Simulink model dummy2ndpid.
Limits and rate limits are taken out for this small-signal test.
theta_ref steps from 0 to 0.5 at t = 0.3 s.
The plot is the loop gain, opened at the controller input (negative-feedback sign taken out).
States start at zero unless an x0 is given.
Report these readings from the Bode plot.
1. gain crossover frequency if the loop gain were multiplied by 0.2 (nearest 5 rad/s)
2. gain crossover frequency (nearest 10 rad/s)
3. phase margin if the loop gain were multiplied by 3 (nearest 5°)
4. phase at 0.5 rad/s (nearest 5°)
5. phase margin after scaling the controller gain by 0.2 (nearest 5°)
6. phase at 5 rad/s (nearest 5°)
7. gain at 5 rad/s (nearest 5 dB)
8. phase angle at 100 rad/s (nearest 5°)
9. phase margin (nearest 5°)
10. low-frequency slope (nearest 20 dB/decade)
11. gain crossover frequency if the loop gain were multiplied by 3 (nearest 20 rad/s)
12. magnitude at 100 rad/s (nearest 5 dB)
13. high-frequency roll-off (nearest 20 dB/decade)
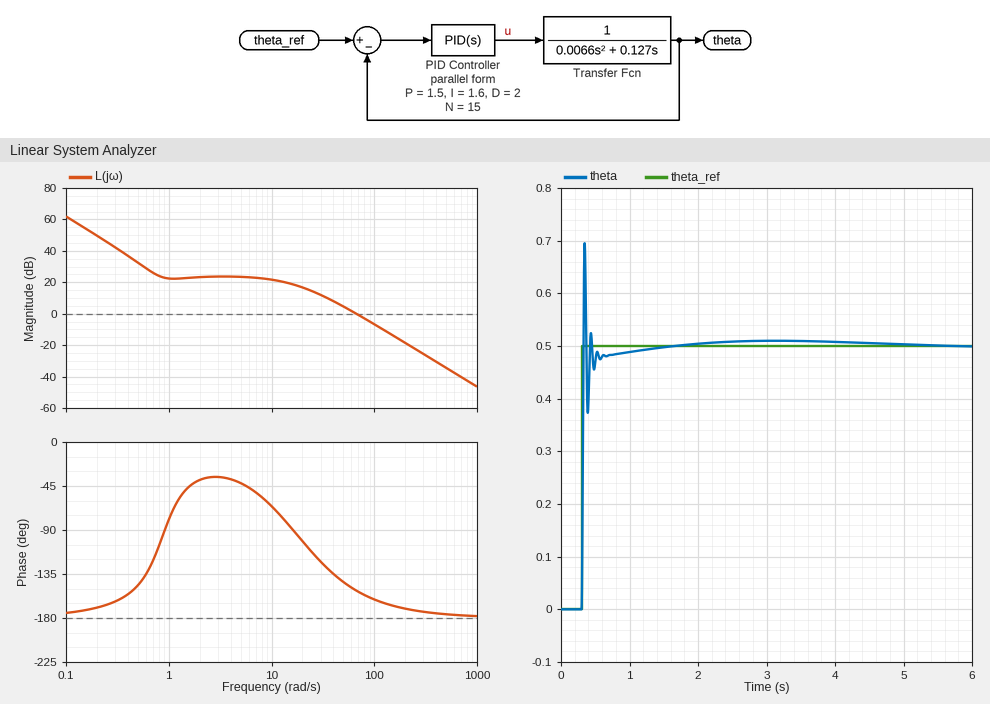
25 rad/s
70 rad/s
15°
-145°
65°
-40°
25 dB
-160°
30°
-40 dB/decade
120 rad/s
-5 dB
-40 dB/decade
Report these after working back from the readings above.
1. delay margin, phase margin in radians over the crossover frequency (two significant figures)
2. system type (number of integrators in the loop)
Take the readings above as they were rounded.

0.0075 s
2
